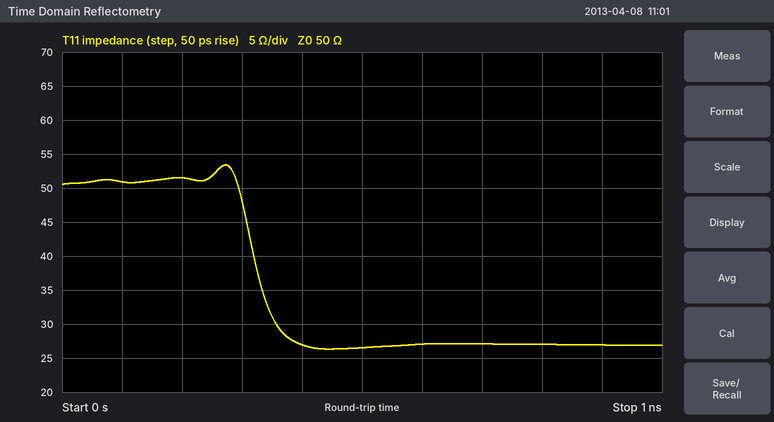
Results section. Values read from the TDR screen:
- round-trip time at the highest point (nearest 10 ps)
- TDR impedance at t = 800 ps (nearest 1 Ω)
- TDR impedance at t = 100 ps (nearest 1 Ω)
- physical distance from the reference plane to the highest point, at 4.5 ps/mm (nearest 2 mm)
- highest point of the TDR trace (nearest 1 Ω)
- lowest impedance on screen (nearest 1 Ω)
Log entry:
270 ps
27 Ω
51 Ω
30 mm
53 Ω
26 Ω
